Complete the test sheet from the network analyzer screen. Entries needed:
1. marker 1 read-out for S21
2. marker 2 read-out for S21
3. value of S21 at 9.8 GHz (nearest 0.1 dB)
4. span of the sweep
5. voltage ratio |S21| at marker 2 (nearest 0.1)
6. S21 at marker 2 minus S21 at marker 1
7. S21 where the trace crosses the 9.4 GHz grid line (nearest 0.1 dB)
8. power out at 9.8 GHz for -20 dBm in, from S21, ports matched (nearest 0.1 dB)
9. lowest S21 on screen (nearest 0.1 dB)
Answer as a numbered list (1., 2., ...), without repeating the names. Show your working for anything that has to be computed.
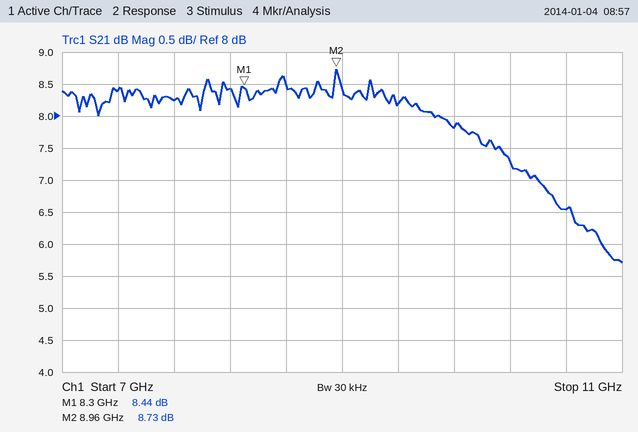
1. 8.44 dB
2. 8.73 dB
3. 7.8 dB
4. 4 GHz
5. 10^(8.73/20) ≈ 2.7
6. 8.73 − (8.44) = 0.29 dB
7. 8.2 dB
8. -20 dBm + (7.8 dB) = -12.2 dBm
9. 5.7 dB
